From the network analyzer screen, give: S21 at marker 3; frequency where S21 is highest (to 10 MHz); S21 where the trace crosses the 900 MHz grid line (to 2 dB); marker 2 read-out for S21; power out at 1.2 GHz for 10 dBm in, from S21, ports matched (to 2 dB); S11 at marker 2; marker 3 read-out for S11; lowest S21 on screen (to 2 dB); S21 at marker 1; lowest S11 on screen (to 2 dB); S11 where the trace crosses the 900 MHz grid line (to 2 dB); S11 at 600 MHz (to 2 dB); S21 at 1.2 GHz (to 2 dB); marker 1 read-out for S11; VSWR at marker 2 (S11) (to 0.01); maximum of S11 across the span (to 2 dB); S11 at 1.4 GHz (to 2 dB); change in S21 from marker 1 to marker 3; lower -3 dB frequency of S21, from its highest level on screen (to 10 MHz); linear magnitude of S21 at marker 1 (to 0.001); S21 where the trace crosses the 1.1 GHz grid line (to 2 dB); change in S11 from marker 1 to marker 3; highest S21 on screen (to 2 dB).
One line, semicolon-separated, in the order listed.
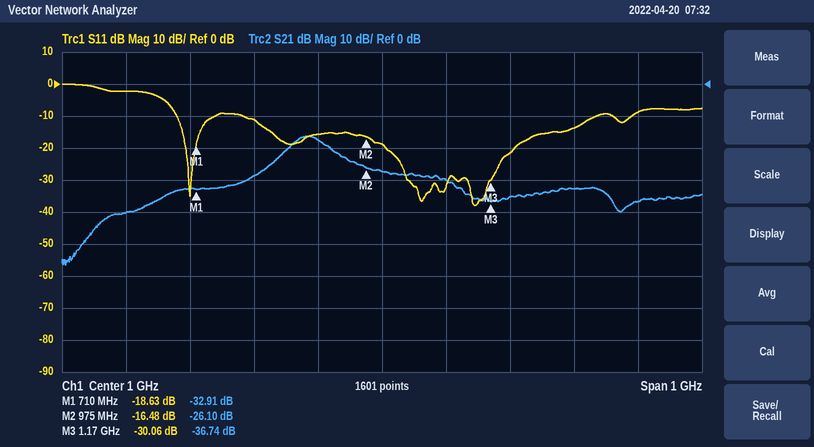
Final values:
-36.74 dB; 880 MHz; -18 dB; -26.10 dB; -26 dBm; -16.48 dB; -30.06 dB; -56 dB; -32.91 dB; -38 dB; -16 dB; -2 dB; -36 dB; -18.63 dB; 1.35; 0 dB; -8 dB; -3.83 dB; 860 MHz; 0.023; -30 dB; -11.43 dB; -16 dB
